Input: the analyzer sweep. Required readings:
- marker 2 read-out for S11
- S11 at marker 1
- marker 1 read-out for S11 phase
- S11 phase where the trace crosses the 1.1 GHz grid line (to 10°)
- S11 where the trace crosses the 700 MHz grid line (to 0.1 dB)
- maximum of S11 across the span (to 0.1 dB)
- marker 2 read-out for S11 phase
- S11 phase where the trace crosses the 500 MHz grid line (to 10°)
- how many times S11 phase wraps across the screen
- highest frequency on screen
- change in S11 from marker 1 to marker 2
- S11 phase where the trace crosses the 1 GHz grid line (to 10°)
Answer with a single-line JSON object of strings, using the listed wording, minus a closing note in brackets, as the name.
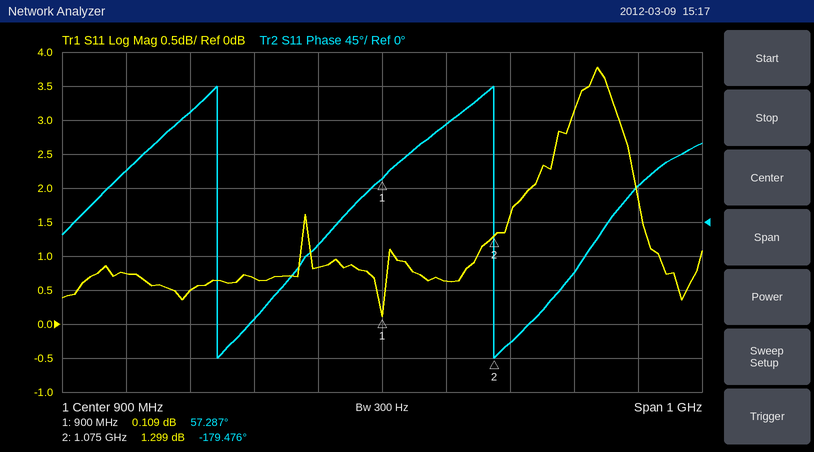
{"marker 2 read-out for S11": "1.299 dB", "S11 at marker 1": "0.109 dB", "marker 1 read-out for S11 phase": "57.287°", "S11 phase where the trace crosses the 1.1 GHz grid line": "-160°", "S11 where the trace crosses the 700 MHz grid line": "0.7 dB", "maximum of S11 across the span": "3.8 dB", "marker 2 read-out for S11 phase": "-179.476°", "S11 phase where the trace crosses the 500 MHz grid line": "70°", "how many times S11 phase wraps across the screen": "2", "highest frequency on screen": "1.4 GHz", "change in S11 from marker 1 to marker 2": "1.190 dB", "S11 phase where the trace crosses the 1 GHz grid line": "130°"}
